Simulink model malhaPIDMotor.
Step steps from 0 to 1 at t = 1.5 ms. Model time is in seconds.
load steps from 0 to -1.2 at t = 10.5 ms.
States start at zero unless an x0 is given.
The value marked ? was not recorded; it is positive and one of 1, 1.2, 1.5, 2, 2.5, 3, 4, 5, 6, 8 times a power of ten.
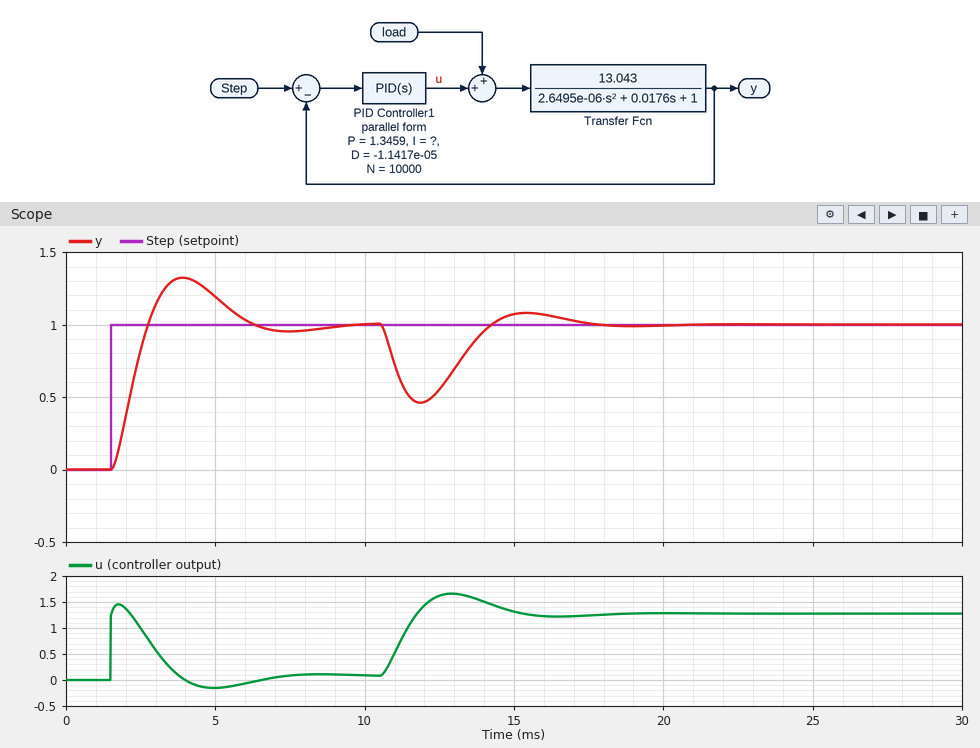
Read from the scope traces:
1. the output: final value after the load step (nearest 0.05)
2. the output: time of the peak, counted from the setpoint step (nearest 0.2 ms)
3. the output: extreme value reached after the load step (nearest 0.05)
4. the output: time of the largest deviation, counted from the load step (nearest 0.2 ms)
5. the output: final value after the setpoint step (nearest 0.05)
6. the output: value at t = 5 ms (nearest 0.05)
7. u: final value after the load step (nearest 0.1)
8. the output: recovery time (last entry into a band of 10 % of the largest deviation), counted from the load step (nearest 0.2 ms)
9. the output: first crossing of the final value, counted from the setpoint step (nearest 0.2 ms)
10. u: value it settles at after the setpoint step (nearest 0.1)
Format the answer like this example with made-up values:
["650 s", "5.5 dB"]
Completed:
["1.00", "2.4 ms", "0.45", "1.4 ms", "1.00", "1.20", "1.3", "5.8 ms", "1.2 ms", "0.1"]
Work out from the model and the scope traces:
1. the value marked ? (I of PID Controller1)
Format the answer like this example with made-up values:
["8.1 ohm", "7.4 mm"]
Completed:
["1200"]
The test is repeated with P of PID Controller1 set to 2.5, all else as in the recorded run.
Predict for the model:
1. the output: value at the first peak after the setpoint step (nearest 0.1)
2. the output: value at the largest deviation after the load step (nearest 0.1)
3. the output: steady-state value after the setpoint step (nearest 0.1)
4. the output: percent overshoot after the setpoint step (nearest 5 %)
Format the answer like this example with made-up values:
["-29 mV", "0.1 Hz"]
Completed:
["1.2", "0.6", "1.0", "15 %"]
